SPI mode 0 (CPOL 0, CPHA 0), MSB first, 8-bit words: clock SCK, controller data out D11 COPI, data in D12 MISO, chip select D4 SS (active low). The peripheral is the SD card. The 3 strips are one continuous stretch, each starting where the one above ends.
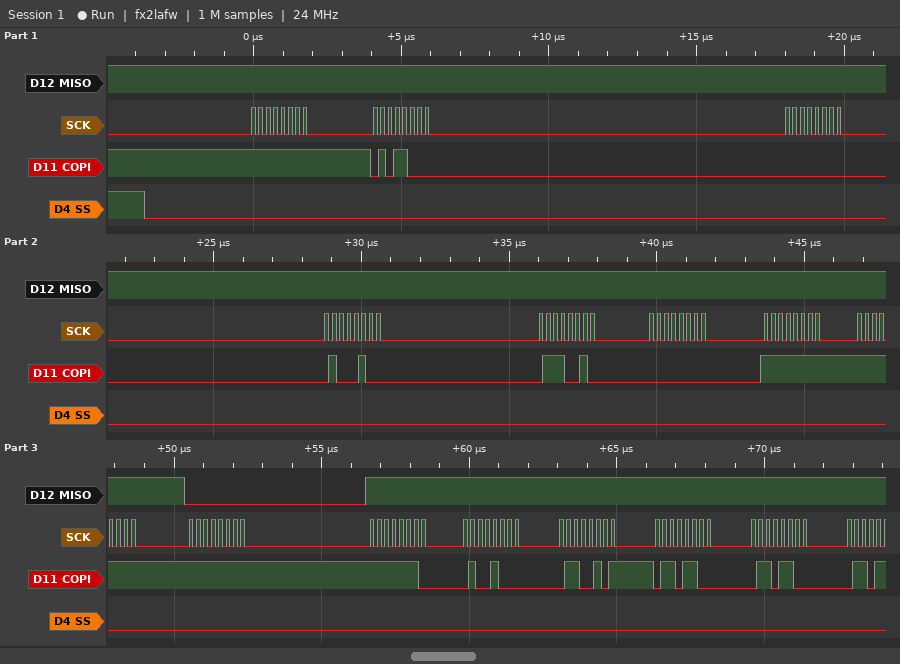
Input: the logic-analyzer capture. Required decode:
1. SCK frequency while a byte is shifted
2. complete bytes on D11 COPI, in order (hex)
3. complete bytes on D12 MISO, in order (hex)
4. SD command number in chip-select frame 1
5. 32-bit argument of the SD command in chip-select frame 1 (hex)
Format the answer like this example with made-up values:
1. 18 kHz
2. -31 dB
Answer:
1. 4 MHz
2. FF 58 00 44 72 00 FF FF FF FE 48 65 6C 6C
3. FF FF FF FF FF FF FF FF 00 FF FF FF FF FF
4. CMD24
5. 0x00447200
